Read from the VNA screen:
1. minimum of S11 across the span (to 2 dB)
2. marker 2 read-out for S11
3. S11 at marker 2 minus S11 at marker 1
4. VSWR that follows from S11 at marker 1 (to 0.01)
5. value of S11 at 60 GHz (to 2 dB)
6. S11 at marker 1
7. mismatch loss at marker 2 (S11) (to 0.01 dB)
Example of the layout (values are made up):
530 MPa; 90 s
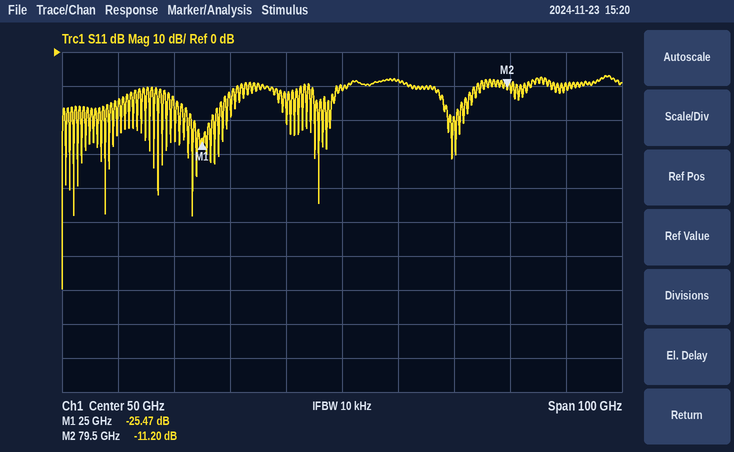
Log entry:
-70 dB; -11.20 dB; 14.27 dB; 1.11; -8 dB; -25.47 dB; 0.34 dB
